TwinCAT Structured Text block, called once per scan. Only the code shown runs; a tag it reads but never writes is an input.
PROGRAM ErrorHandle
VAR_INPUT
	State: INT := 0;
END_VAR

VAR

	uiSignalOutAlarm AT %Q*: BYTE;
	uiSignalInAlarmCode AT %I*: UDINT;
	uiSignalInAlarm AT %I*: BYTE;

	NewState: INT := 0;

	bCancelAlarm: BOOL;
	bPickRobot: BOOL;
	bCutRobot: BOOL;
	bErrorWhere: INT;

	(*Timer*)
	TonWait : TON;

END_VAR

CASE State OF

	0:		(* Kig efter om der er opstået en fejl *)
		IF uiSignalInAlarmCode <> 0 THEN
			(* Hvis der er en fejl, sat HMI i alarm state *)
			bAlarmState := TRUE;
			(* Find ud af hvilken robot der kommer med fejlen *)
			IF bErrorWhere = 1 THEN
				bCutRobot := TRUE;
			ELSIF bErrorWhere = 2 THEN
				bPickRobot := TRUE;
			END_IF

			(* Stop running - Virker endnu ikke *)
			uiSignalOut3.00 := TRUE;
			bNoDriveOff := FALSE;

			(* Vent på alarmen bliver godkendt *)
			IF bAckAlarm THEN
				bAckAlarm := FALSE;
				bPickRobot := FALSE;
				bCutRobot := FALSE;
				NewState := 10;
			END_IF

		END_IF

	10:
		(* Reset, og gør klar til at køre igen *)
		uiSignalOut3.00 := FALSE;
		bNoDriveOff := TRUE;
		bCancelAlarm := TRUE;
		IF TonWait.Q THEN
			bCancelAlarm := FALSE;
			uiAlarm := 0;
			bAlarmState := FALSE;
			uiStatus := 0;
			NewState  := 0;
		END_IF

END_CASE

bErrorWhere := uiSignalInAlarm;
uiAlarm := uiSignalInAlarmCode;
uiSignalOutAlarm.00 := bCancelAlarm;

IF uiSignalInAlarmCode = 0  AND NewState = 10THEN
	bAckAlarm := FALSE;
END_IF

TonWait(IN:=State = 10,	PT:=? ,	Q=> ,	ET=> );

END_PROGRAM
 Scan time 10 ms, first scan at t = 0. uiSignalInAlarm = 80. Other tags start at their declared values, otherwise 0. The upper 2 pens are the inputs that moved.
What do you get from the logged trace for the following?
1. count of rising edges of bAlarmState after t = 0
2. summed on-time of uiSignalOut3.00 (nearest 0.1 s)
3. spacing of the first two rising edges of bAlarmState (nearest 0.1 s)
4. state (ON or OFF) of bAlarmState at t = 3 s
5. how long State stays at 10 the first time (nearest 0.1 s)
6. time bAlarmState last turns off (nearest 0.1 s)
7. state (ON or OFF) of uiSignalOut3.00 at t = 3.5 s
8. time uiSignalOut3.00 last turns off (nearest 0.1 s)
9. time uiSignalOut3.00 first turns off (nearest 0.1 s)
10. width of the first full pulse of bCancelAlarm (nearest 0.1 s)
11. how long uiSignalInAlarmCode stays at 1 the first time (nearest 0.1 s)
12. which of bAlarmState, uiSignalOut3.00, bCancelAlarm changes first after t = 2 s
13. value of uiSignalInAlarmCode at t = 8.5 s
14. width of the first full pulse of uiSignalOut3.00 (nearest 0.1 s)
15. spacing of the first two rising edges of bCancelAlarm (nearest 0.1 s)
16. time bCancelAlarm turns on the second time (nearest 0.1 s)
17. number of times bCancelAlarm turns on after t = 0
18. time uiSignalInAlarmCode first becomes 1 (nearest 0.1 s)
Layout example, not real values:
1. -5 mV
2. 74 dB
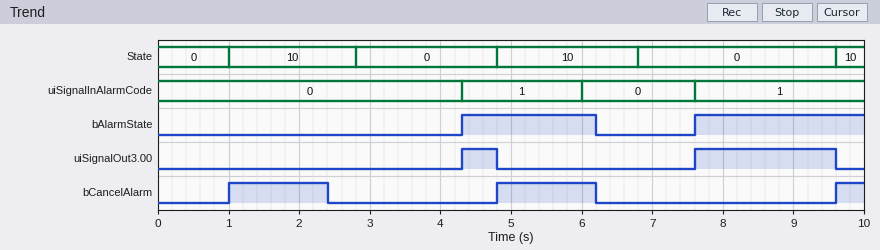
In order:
1. 2
2. 2.5 s
3. 3.3 s
4. OFF
5. 1.8 s
6. 6.2 s
7. OFF
8. 9.6 s
9. 4.8 s
10. 1.4 s
11. 1.7 s
12. bCancelAlarm
13. 1
14. 0.5 s
15. 3.8 s
16. 4.8 s
17. 3
18. 4.3 s
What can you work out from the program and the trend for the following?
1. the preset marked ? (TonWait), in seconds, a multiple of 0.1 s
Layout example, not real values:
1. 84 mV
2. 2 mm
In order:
1. 1.4 s
